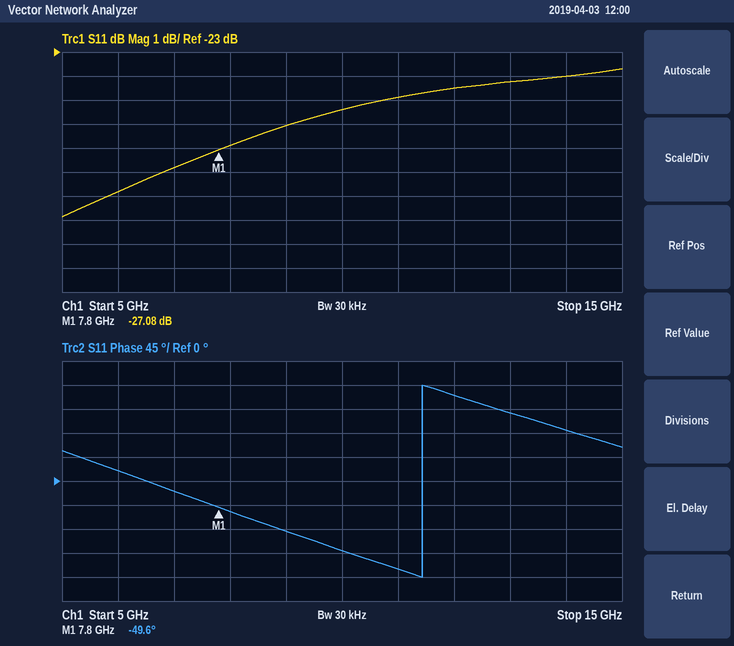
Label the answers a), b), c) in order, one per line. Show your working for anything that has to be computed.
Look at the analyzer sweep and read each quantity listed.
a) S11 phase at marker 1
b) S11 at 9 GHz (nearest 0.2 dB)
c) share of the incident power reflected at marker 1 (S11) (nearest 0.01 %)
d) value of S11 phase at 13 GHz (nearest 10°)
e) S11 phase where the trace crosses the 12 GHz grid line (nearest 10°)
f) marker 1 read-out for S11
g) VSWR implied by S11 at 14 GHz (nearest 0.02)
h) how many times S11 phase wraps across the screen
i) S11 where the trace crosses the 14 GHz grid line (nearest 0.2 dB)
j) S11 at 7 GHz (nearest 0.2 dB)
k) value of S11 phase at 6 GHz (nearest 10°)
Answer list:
a) -49.6°
b) -26.0 dB
c) 10^(-27.08/10) ≈ 0.20 %
d) 130°
e) 160°
f) -27.08 dB
g) |Γ| = 10^(-24/20) = 0.0631; VSWR = (1 + 0.0631)/(1 − 0.0631) ≈ 1.13, so 1.14 to the nearest 0.02
h) 1
i) -24.0 dB
j) -27.8 dB
k) 20°
